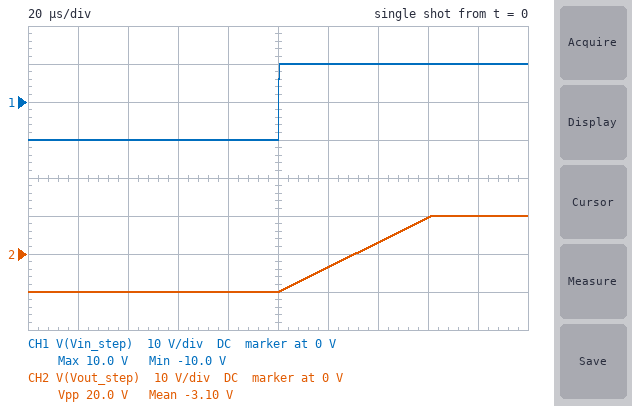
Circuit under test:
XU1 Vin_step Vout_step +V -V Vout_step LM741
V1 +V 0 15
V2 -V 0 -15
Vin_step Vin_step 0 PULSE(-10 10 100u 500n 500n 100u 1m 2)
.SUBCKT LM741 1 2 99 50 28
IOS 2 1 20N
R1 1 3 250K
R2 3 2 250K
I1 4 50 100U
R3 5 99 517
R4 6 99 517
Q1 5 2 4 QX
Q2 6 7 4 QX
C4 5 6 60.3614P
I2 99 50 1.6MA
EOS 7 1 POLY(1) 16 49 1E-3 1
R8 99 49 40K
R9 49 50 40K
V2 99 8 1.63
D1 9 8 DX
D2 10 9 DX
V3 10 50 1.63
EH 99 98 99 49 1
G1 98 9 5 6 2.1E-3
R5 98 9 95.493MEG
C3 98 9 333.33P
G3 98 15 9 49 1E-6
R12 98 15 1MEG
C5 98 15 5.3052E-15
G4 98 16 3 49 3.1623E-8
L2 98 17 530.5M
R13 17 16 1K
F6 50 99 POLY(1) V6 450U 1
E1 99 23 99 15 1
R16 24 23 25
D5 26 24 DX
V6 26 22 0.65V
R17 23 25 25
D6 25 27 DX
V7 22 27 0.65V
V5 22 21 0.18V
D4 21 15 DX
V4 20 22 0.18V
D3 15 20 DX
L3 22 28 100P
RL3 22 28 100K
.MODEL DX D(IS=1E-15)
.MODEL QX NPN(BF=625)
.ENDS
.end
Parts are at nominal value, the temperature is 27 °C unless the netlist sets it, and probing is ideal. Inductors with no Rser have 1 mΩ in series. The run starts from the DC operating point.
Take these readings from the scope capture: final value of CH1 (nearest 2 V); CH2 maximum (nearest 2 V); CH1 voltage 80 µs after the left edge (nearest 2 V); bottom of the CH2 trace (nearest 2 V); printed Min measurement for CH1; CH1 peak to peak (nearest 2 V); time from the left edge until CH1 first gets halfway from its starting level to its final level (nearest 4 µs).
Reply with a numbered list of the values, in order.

1. 10 V
2. 10 V
3. -10 V
4. -10 V
5. -10.0 V
6. 20 V
7. 100 µs
